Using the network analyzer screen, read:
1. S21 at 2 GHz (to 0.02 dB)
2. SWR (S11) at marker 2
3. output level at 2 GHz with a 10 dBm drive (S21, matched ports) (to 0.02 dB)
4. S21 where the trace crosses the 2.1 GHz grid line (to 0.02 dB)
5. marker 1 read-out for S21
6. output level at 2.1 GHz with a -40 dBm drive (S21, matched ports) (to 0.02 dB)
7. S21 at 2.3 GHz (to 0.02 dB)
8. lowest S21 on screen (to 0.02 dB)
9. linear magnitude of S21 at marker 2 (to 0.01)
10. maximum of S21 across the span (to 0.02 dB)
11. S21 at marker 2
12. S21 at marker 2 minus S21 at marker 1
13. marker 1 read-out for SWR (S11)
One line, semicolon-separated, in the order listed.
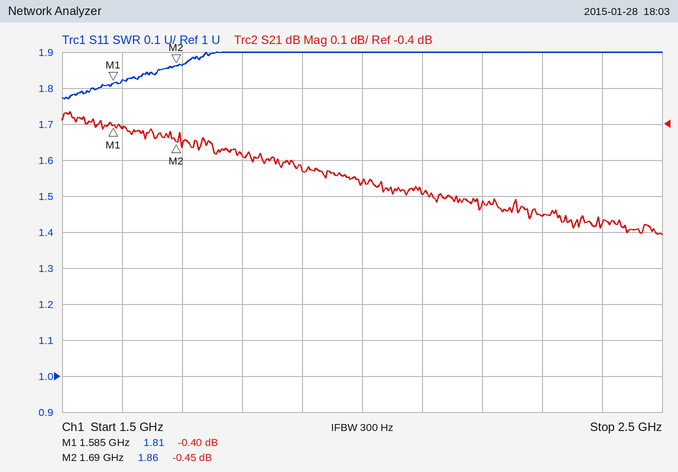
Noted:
-0.56 dB; 1.86; 9.44 dBm; -0.60 dB; -0.40 dB; -40.60 dBm; -0.66 dB; -0.70 dB; 0.95; -0.36 dB; -0.45 dB; -0.05 dB; 1.81
